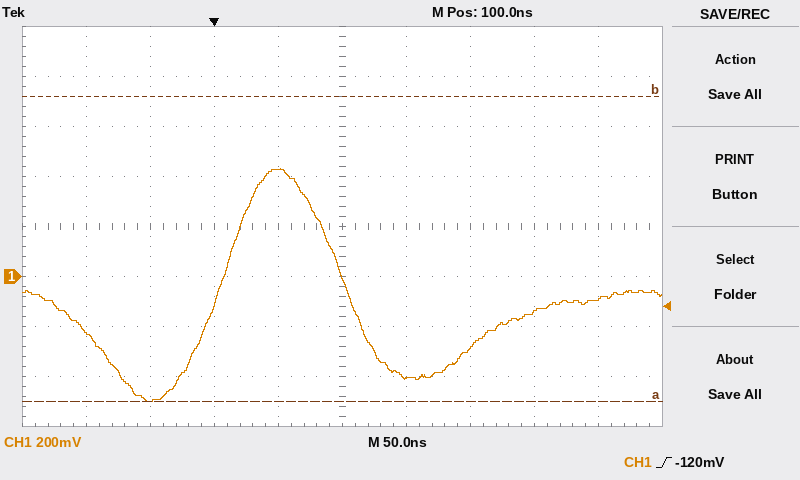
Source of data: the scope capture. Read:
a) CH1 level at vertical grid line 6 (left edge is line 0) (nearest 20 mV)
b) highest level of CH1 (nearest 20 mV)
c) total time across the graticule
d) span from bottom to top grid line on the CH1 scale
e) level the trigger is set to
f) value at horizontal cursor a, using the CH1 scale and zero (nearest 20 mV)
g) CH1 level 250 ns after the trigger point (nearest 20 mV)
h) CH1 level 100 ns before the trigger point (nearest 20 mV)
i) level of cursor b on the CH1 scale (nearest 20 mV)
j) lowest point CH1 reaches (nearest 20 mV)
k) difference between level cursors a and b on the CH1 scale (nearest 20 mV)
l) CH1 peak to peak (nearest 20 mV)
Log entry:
-400 mV
440 mV
500 ns
1.6 V
-120 mV
-500 mV
-140 mV
-220 mV
720 mV
-500 mV
1.22 V
940 mV
